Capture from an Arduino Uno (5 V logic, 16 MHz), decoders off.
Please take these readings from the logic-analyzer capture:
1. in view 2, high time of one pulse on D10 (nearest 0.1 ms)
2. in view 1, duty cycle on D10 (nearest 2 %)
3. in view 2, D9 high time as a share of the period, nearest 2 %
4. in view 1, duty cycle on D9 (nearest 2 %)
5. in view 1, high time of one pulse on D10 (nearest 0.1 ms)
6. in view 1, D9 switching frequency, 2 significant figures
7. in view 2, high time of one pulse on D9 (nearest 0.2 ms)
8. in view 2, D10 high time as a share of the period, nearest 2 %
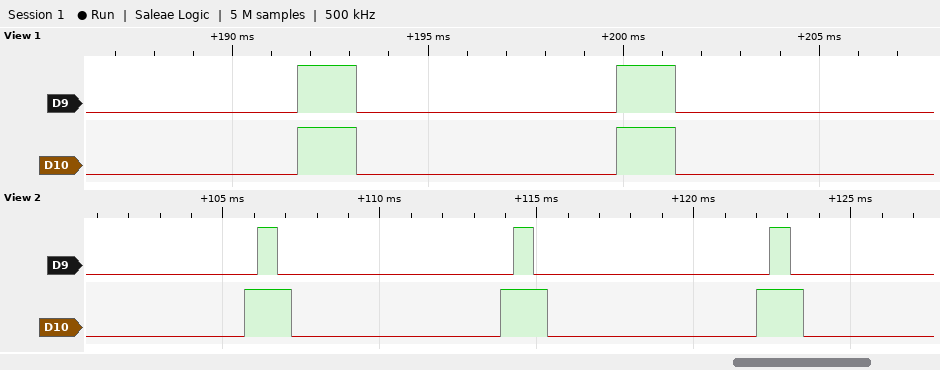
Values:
1.5 ms
18 %
8 %
18 %
1.5 ms
120 Hz
0.6 ms
18 %
